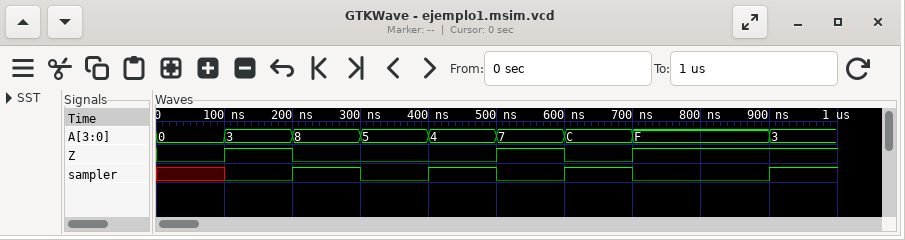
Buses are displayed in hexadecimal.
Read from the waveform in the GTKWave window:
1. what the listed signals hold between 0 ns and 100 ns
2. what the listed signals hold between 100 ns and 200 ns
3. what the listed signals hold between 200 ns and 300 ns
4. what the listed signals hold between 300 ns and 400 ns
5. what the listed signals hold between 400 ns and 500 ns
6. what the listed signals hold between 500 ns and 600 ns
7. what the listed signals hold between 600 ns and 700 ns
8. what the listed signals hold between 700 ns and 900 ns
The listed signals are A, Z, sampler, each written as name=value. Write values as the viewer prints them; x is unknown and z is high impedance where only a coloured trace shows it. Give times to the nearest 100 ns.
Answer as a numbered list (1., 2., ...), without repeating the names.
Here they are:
1. A=0, Z=0, sampler=x
2. A=3, Z=1, sampler=0
3. A=8, Z=0, sampler=1
4. A=5, Z=0, sampler=0
5. A=4, Z=0, sampler=1
6. A=7, Z=1, sampler=0
7. A=C, Z=0, sampler=1
8. A=F, Z=1, sampler=0
